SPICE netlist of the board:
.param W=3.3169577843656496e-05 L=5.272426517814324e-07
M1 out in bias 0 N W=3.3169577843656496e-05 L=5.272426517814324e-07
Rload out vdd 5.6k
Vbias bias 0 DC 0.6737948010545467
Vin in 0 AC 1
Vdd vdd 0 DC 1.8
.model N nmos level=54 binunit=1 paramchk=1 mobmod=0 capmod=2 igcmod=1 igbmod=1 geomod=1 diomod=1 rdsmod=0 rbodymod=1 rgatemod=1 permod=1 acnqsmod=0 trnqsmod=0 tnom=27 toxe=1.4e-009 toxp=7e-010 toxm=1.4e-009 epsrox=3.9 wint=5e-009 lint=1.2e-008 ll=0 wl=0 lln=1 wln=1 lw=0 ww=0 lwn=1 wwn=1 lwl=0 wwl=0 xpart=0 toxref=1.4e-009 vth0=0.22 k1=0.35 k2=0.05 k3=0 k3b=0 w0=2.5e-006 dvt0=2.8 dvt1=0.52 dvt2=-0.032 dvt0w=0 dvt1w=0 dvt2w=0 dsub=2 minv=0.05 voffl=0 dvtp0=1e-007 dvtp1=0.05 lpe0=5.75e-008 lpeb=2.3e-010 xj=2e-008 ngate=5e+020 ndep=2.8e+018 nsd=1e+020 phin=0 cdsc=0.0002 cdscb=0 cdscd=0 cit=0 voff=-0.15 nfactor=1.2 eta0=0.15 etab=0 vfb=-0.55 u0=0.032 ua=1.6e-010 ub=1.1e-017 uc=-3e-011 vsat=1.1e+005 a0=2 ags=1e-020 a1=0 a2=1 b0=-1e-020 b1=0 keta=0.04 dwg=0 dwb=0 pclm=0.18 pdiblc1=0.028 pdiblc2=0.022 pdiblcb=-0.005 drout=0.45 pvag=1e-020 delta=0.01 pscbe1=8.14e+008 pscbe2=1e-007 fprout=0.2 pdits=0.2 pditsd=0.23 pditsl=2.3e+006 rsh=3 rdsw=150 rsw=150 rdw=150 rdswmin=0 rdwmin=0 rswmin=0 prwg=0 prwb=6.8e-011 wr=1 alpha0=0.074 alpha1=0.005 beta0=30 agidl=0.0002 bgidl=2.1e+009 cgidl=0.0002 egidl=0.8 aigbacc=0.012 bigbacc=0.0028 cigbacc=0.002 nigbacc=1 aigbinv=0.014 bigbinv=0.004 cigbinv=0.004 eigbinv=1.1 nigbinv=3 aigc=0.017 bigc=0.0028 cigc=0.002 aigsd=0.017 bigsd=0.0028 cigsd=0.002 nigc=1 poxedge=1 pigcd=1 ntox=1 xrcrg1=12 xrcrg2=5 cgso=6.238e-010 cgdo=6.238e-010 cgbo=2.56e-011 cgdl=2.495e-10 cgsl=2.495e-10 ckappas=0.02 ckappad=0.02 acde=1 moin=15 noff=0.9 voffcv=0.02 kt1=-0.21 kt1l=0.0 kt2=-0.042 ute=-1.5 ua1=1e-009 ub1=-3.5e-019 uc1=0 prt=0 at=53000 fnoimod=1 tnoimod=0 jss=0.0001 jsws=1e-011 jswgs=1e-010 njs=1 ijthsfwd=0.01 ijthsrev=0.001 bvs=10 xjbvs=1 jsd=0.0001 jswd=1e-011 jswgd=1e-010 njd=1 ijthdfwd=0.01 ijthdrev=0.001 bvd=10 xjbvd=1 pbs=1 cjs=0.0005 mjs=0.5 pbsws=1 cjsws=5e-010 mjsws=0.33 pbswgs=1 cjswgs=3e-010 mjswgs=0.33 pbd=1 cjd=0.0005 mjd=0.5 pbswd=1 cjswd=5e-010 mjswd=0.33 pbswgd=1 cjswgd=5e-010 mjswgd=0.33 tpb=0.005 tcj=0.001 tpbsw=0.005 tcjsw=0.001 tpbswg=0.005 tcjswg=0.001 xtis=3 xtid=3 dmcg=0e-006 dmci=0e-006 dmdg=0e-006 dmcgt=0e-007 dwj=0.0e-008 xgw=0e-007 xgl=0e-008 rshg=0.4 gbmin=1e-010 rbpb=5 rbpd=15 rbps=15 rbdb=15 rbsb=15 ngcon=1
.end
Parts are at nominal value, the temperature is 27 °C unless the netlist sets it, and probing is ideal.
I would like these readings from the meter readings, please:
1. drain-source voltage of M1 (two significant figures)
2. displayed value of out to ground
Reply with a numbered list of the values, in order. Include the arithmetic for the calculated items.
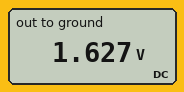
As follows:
1. 1.627 V - 673.8 mV = 950 mV
2. 1.627 V
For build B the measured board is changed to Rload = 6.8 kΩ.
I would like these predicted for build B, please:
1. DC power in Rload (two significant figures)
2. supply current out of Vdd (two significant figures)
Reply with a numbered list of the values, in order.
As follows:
1. 4.9 µW
2. 27 µA
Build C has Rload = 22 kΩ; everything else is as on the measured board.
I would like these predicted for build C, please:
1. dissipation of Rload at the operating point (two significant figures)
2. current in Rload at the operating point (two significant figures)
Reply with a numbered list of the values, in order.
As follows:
1. 2.7 µW
2. 11 µA
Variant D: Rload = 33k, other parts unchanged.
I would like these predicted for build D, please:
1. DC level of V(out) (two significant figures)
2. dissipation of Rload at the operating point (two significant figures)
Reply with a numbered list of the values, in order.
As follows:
1. 1.5 V
2. 2.1 µW
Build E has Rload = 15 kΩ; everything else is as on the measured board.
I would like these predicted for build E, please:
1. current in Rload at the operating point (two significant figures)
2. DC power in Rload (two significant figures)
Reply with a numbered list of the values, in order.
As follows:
1. 15 µA
2. 3.3 µW
